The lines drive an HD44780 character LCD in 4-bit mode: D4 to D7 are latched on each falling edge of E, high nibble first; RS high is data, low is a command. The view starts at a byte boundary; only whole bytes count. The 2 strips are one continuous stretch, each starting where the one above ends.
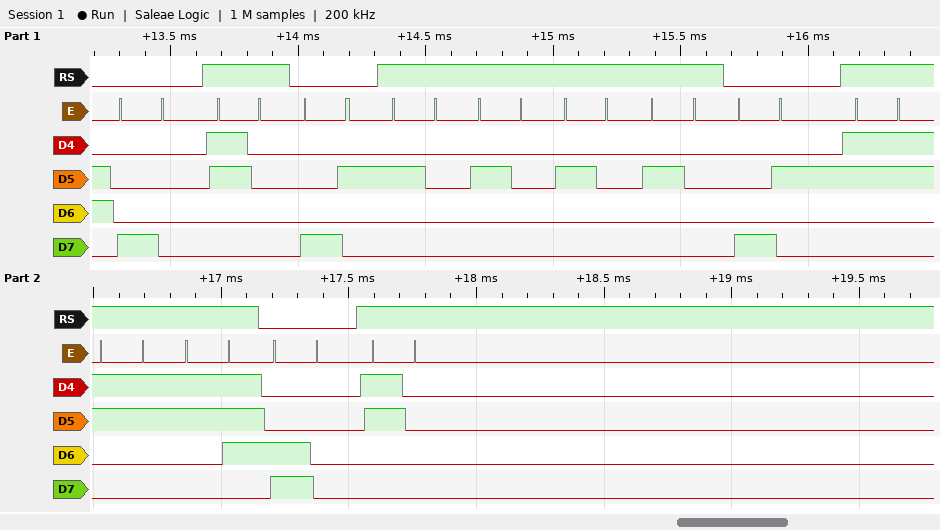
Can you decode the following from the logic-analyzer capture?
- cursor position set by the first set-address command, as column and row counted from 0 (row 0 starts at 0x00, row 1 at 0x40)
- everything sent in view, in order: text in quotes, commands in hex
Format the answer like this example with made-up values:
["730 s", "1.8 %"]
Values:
["column 0, row 0", "0x80 \"0\" 0x82 \"    \" 0x82 \"337\" 0xC0 \"0\""]
